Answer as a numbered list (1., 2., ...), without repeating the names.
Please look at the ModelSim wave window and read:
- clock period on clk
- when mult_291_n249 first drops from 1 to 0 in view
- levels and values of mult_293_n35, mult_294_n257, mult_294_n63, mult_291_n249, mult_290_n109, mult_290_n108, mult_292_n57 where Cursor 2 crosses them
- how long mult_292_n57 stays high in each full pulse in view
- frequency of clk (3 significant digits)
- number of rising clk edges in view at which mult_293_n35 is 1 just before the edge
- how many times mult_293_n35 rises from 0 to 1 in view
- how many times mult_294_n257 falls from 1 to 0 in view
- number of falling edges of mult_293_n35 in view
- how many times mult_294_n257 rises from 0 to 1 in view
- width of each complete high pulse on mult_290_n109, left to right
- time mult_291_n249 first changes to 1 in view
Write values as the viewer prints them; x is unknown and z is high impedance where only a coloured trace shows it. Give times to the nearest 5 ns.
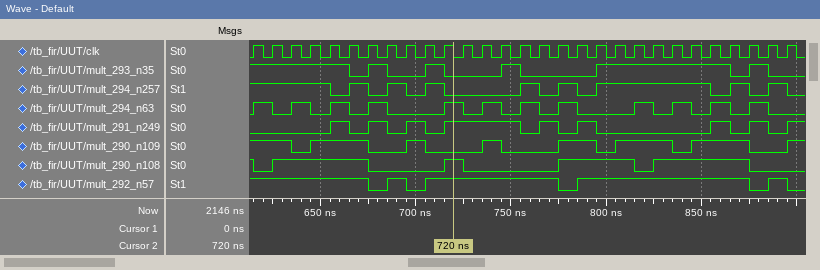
1. 10 ns
2. 665 ns
3. mult_293_n35=0, mult_294_n257=0, mult_294_n63=1, mult_291_n249=1, mult_290_n109=0, mult_290_n108=1, mult_292_n57=1
4. 10 ns, 70 ns, 90 ns, 10 ns
5. 100 MHz
6. 17
7. 5
8. 9
9. 6
10. 8
11. 30 ns, 10 ns, 10 ns, 20 ns, 30 ns, 30 ns
12. 655 ns
